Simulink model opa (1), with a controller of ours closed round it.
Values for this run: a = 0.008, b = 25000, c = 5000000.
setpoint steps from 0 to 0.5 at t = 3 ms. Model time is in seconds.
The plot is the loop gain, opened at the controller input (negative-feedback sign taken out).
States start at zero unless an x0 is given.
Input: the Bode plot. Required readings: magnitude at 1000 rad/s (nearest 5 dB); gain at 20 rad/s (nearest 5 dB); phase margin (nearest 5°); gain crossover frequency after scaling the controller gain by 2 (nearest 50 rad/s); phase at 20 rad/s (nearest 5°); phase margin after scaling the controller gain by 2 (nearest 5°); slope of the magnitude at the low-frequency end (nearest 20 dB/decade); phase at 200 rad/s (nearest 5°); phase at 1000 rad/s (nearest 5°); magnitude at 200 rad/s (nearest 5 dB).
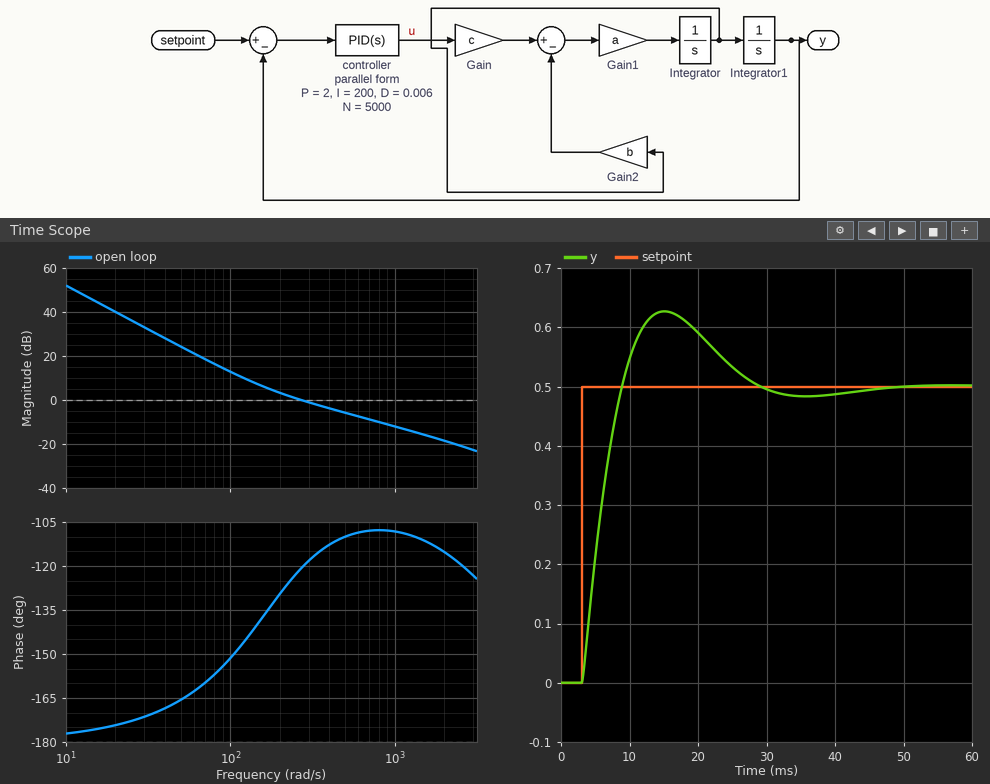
-10 dB
40 dB
60°
500 rad/s
-175°
70°
-40 dB/decade
-130°
-110°
5 dB
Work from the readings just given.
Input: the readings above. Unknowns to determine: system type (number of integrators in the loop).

2
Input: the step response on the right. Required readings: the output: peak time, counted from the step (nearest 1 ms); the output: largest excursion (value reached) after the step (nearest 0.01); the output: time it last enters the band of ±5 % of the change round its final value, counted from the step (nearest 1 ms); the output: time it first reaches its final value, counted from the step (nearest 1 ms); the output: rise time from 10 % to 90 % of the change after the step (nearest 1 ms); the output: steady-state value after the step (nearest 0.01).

12 ms
0.63
23 ms
6 ms
4 ms
0.50
